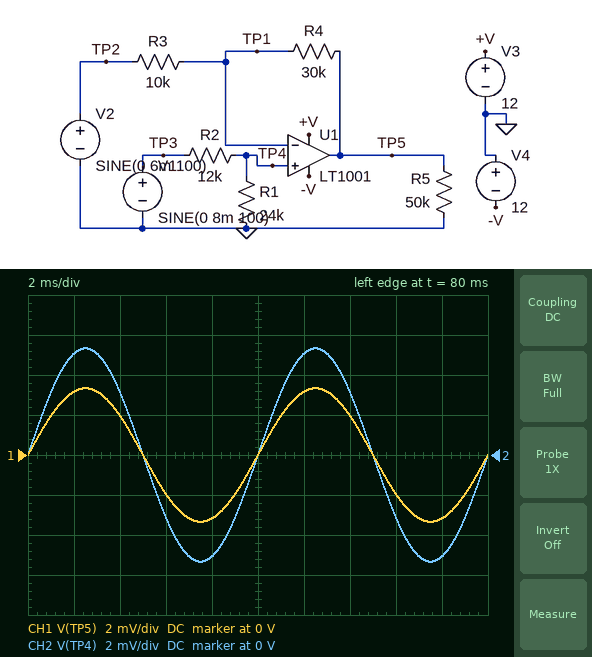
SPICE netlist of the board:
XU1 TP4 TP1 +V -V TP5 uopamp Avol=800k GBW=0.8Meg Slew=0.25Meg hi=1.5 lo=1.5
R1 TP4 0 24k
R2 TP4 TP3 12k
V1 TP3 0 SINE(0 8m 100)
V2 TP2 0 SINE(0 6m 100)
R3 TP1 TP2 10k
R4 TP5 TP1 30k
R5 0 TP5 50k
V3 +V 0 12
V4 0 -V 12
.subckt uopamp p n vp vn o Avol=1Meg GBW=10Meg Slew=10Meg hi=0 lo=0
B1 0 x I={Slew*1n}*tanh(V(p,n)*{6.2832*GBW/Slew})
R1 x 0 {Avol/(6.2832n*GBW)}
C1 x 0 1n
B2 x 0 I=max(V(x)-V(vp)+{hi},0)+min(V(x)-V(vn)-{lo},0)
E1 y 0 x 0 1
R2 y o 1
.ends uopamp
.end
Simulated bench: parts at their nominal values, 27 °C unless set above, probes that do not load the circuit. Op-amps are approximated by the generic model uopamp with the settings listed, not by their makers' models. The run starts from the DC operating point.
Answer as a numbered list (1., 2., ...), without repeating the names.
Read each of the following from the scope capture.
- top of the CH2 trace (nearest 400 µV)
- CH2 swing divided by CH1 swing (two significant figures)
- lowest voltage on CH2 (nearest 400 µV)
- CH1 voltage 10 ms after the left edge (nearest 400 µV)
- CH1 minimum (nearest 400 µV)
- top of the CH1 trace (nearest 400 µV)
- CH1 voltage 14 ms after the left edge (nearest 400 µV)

1. 5.2 mV
2. 1.6
3. -5.2 mV
4. 0 V
5. -3.2 mV
6. 3.2 mV
7. 2.0 mV
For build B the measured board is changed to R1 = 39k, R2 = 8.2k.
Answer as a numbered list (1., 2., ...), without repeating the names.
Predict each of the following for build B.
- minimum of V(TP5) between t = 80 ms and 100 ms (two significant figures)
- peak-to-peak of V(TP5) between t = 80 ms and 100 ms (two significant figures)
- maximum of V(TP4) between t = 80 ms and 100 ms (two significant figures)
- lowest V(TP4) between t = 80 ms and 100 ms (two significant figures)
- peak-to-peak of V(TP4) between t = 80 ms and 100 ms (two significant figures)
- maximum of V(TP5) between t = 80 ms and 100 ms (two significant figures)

1. -8.4 mV
2. 17 mV
3. 6.6 mV
4. -6.6 mV
5. 13 mV
6. 8.4 mV
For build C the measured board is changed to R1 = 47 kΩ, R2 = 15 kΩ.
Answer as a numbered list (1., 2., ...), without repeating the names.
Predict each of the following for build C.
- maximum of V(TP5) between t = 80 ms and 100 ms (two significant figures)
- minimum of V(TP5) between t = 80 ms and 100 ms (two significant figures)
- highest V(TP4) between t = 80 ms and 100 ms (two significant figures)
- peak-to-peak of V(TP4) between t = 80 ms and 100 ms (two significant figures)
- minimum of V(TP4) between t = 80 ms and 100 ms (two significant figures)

1. 6.3 mV
2. -6.3 mV
3. 6.1 mV
4. 12 mV
5. -6.1 mV
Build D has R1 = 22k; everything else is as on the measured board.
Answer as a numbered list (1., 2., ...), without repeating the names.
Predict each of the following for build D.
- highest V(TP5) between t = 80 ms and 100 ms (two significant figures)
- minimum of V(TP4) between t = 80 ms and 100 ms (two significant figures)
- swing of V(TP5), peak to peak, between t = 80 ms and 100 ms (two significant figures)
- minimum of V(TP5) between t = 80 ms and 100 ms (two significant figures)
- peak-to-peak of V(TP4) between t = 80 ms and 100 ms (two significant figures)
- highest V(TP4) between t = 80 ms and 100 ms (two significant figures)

1. 2.7 mV
2. -5.2 mV
3. 5.4 mV
4. -2.7 mV
5. 10 mV
6. 5.2 mV
